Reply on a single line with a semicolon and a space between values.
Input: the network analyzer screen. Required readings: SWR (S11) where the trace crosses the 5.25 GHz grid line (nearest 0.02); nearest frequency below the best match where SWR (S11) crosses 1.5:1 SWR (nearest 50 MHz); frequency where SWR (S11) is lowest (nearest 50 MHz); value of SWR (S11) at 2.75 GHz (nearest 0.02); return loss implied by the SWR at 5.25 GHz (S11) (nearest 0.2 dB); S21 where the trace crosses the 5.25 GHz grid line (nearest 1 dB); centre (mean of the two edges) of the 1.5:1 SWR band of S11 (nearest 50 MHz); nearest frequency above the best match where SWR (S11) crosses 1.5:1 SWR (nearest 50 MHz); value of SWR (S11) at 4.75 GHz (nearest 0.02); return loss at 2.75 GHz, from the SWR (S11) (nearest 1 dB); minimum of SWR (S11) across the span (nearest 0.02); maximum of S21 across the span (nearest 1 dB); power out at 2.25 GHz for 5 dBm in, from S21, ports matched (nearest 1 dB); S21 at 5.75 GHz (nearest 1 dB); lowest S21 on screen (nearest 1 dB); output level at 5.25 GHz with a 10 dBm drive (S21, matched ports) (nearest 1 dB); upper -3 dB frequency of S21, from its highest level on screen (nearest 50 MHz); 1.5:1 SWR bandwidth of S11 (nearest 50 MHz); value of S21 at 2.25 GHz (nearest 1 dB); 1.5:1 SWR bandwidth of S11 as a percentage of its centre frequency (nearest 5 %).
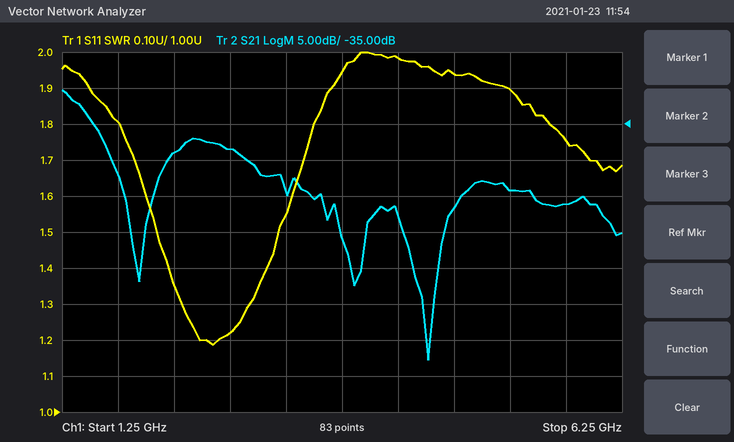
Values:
1.90; 2.10 GHz; 2.60 GHz; 1.22; 10.2 dB; -44 dB; 2.65 GHz; 3.20 GHz; 1.94; 20 dB; 1.18; -30 dB; -34 dBm; -46 dB; -68 dB; -34 dBm; 1.45 GHz; 1.10 GHz; -39 dB; 40 %
